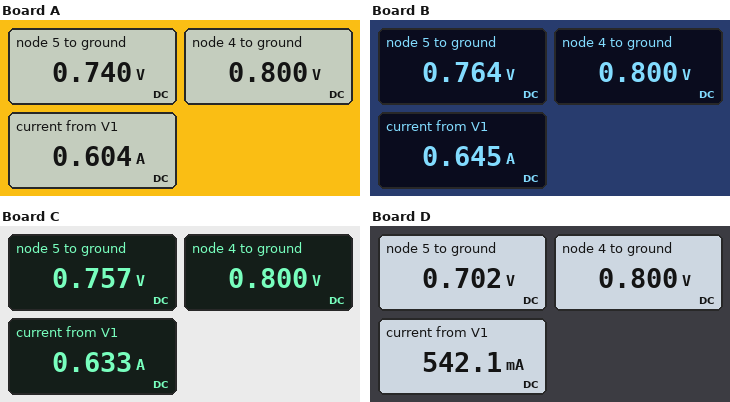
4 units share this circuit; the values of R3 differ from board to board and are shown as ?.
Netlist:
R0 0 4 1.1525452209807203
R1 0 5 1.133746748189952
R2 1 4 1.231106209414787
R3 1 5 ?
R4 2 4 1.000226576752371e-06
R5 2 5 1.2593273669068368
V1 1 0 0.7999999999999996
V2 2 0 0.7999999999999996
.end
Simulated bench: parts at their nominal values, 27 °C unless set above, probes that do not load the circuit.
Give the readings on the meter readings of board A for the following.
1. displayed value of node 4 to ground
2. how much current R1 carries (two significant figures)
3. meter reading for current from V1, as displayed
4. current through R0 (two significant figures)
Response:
0.800 V
650 mA
0.604 A
690 mA
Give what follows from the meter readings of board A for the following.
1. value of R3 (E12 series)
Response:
0.1 Ω
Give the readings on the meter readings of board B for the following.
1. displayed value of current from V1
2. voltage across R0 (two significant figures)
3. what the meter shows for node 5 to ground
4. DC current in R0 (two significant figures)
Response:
0.645 A
800 mV
0.764 V
690 mA
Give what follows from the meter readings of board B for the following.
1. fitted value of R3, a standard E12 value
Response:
0.056 Ω
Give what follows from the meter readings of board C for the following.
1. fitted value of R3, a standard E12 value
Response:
0.068 Ω
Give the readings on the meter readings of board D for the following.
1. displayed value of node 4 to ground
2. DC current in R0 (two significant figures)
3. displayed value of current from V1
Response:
0.800 V
690 mA
542.1 mA
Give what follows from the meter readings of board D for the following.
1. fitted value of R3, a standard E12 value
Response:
0.18 Ω
